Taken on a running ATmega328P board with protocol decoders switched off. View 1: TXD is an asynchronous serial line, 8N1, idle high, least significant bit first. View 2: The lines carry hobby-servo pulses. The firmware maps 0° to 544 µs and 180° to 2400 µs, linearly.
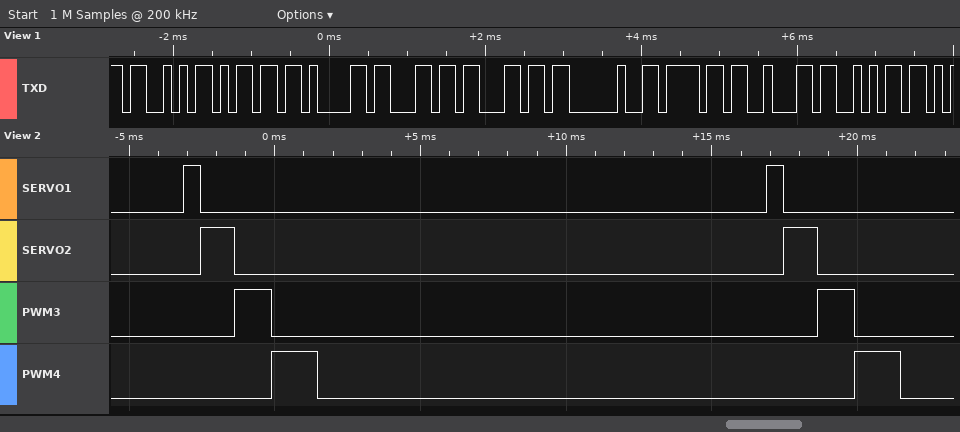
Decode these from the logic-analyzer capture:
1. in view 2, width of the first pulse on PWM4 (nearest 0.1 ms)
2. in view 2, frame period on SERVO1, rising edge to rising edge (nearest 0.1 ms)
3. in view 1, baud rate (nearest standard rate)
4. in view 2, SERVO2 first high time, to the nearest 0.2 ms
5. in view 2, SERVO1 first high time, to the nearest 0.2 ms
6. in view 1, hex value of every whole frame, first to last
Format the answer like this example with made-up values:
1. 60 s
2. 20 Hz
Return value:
1. 1.6 ms
2. 20.0 ms
3. 9600 baud
4. 1.2 ms
5. 0.6 ms
6. 53 6D 61 6C 6C 20 6F 62 6A
